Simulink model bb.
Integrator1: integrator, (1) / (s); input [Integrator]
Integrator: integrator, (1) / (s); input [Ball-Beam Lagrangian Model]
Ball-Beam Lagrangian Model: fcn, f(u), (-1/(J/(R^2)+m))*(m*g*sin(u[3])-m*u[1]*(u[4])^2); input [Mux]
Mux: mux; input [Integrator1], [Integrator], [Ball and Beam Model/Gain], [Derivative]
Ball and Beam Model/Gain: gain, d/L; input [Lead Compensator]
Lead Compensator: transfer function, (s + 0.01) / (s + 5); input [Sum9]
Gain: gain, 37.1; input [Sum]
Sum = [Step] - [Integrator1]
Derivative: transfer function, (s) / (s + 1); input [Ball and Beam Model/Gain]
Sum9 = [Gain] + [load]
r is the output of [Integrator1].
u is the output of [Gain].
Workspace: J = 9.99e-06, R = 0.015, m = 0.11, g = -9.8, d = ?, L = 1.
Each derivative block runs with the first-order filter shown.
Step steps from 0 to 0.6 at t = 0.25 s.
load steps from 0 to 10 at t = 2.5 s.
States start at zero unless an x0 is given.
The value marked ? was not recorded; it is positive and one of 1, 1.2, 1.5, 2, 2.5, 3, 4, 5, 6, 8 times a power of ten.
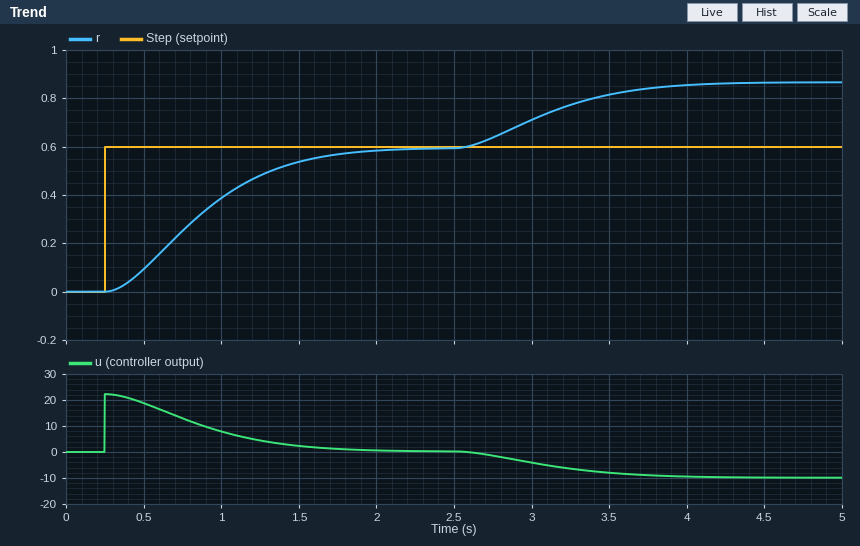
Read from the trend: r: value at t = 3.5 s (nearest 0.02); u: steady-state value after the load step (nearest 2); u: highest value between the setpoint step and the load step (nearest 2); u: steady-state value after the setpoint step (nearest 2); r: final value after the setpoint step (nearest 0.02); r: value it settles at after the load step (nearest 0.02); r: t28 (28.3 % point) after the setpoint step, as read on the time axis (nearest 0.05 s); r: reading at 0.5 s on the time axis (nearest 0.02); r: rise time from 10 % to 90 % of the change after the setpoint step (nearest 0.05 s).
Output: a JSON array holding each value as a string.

["0.82", "-10", "22", "0", "0.60", "0.86", "0.60 s", "0.10", "1.05 s"]
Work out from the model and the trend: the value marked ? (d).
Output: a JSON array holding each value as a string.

["0.03"]
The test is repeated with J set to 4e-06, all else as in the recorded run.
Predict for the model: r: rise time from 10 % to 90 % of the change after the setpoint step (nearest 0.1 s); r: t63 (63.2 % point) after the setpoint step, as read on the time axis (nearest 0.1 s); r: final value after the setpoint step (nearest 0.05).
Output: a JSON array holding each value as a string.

["0.8 s", "0.9 s", "0.60"]
